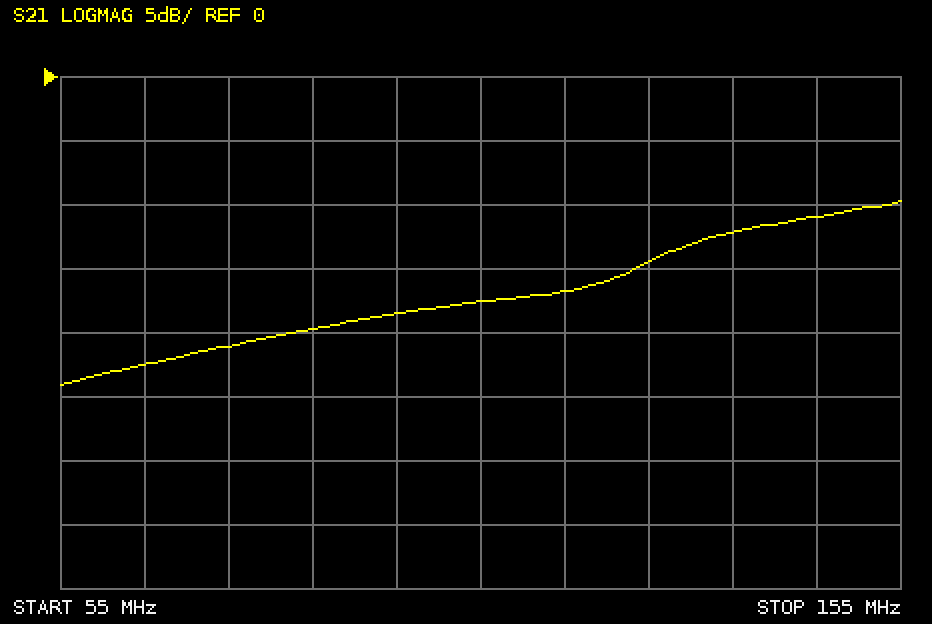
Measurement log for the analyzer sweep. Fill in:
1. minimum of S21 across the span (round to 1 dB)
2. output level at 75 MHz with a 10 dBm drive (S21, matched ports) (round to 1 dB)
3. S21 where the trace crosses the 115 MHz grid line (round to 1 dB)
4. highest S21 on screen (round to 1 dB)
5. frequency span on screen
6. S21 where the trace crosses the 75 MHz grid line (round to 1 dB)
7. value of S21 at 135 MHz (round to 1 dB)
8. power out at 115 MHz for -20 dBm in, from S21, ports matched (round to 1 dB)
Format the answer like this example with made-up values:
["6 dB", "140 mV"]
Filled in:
["-24 dB", "-11 dBm", "-17 dB", "-10 dB", "100 MHz", "-21 dB", "-12 dB", "-37 dBm"]
